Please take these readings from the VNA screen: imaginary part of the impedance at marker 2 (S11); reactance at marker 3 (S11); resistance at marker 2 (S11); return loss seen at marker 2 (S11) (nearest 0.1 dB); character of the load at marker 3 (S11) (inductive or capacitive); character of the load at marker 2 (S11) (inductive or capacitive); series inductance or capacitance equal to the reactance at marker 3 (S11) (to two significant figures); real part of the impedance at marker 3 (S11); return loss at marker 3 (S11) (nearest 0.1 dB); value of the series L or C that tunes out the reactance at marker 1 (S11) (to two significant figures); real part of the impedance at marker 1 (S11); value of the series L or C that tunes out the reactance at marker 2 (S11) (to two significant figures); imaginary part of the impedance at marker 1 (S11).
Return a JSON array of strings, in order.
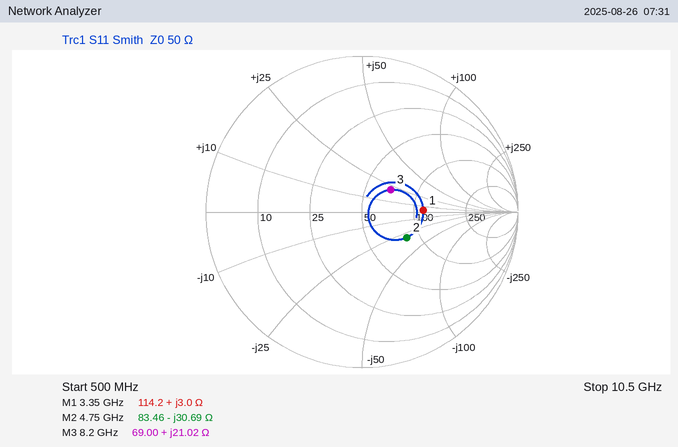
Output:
["-30.69 Ω", "+21.02 Ω", "83.46 Ω", "9.6 dB", "inductive", "capacitive", "410 pH", "69.00 Ω", "12.6 dB", "16 pF", "114.2 Ω", "1.0 nH", "+3.0 Ω"]
